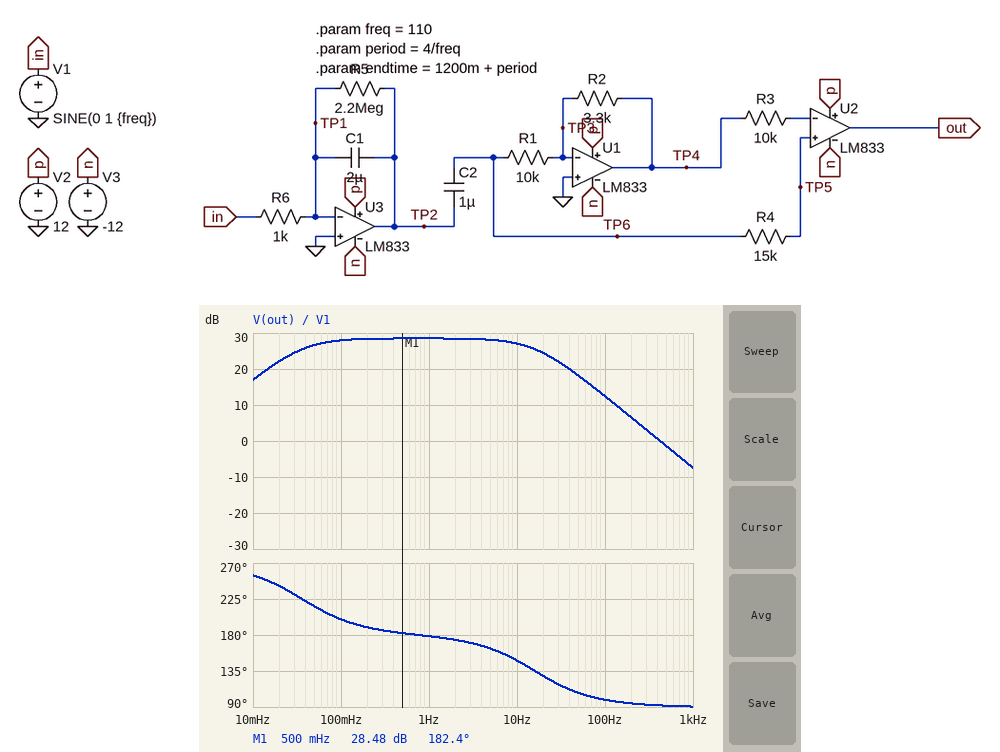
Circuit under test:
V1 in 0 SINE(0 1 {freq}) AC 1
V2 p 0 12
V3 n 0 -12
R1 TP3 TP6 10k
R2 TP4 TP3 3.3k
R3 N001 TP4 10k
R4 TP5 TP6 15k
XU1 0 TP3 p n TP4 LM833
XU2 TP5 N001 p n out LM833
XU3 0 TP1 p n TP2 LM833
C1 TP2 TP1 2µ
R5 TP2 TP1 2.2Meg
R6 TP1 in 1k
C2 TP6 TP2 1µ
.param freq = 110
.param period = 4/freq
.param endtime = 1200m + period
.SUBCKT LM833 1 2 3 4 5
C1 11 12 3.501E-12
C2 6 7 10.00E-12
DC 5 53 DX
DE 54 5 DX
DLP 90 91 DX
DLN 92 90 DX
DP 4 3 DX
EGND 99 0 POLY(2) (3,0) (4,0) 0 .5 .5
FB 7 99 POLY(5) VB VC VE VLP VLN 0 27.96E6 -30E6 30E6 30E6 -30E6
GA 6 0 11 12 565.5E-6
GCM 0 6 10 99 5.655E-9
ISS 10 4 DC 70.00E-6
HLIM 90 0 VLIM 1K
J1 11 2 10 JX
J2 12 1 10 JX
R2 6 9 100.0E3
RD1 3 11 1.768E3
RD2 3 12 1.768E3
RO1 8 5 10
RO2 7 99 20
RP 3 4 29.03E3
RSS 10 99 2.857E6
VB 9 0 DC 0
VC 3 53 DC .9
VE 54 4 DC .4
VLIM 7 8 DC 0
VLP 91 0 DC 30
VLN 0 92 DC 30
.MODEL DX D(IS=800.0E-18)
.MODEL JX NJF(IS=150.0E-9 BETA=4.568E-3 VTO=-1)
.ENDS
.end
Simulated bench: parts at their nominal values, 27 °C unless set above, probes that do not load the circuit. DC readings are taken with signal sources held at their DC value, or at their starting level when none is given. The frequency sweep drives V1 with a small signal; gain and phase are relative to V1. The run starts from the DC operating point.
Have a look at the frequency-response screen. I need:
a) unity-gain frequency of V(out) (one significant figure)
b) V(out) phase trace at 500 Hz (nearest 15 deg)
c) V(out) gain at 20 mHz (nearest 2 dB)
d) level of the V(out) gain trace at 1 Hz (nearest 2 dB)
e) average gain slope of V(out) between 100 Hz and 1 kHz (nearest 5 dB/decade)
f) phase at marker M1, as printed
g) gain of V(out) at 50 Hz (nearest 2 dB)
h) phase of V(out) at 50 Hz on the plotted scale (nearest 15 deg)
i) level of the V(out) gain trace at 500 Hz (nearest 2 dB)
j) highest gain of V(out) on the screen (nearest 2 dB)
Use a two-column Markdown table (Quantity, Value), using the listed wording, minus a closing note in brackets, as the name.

| Quantity | Value |
|---|---|
| unity-gain frequency of V(out) | 400 Hz |
| V(out) phase trace at 500 Hz | 90 deg |
| V(out) gain at 20 mHz | 22 dB |
| level of the V(out) gain trace at 1 Hz | 28 dB |
| average gain slope of V(out) between 100 Hz and 1 kHz | -20 dB/decade |
| phase at marker M1, as printed | 182.4 deg |
| gain of V(out) at 50 Hz | 18 dB |
| phase of V(out) at 50 Hz on the plotted scale | 105 deg |
| level of the V(out) gain trace at 500 Hz | -2 dB |
| highest gain of V(out) on the screen | 28 dB |
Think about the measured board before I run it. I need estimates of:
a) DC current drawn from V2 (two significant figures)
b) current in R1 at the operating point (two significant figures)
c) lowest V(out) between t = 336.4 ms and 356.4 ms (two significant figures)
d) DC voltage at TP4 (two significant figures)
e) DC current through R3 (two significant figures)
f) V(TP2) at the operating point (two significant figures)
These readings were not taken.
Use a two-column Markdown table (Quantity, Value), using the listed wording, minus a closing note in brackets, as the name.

| Quantity | Value |
|---|---|
| DC current drawn from V2 | 2.7 mA |
| current in R1 at the operating point | 300 nA |
| lowest V(out) between t = 336.4 ms and 356.4 ms | -12 V |
| DC voltage at TP4 | -2.0 mV |
| DC current through R3 | 300 nA |
| V(TP2) at the operating point | -670 mV |
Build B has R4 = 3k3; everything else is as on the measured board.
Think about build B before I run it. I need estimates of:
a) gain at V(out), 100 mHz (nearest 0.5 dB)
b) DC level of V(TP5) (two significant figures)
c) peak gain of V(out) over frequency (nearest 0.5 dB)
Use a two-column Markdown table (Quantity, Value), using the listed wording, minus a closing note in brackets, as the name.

| Quantity | Value |
|---|---|
| gain at V(out), 100 mHz | 35.0 dB |
| DC level of V(TP5) | 4.0 mV |
| peak gain of V(out) over frequency | 35.5 dB |
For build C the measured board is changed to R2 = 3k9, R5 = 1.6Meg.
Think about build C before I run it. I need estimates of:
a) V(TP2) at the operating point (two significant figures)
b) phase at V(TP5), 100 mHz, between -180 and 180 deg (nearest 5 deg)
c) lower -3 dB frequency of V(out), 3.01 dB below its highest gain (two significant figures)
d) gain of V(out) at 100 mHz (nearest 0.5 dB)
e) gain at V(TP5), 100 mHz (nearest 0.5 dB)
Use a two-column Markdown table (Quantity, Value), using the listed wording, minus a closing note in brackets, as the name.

| Quantity | Value |
|---|---|
| V(TP2) at the operating point | -490 mV |
| phase at V(TP5), 100 mHz, between -180 and 180 deg | -155 deg |
| lower -3 dB frequency of V(out), 3.01 dB below its highest gain | 50 mHz |
| gain of V(out) at 100 mHz | 27.5 dB |
| gain at V(TP5), 100 mHz | 13.0 dB |
